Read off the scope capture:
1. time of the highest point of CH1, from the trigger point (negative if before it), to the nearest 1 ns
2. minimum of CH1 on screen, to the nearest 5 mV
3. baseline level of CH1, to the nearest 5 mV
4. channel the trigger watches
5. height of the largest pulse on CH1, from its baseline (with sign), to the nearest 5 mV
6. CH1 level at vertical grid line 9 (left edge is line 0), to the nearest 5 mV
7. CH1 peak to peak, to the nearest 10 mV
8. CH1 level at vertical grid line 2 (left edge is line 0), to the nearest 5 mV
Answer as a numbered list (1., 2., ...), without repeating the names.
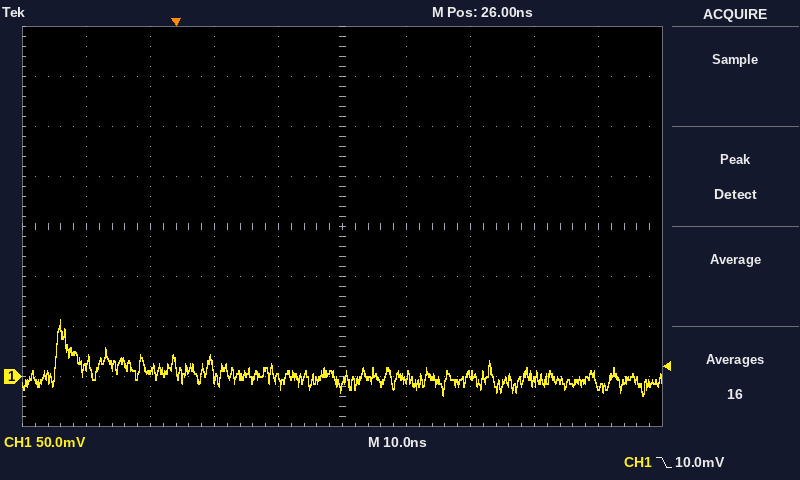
1. -18 ns
2. -20 mV
3. 0 mV
4. CH1
5. +60 mV
6. -10 mV
7. 80 mV
8. 5 mV
